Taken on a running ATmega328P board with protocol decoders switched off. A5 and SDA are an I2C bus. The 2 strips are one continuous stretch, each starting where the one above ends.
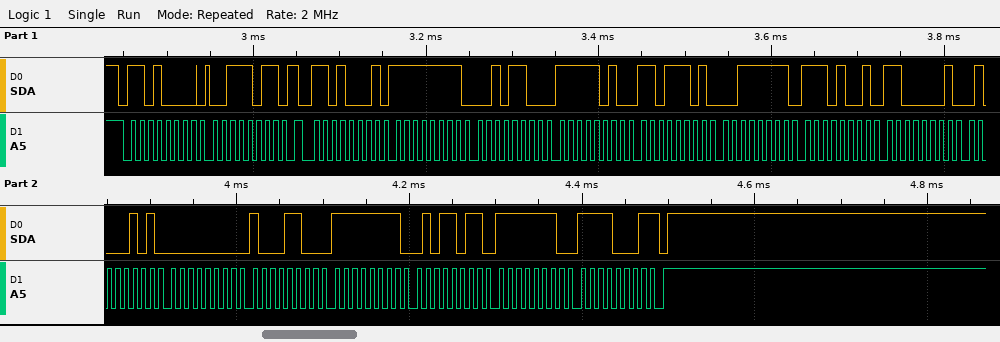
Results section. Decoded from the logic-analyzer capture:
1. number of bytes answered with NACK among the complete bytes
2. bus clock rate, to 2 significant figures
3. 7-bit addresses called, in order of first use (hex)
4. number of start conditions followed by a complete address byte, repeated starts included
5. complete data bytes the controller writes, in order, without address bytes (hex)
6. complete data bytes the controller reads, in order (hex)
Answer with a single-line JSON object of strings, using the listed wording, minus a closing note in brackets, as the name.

{"number of bytes answered with NACK among the complete bytes": "1", "bus clock rate, to 2 significant figures": "100 kHz", "7-bit addresses called, in order of first use": "0x68", "number of start conditions followed by a complete address byte, repeated starts included": "2", "complete data bytes the controller writes, in order, without address bytes": "3B", "complete data bytes the controller reads, in order": "FF 2C FA DD 3F E9 C1 45 00 8C FF 5B FE F1"}
